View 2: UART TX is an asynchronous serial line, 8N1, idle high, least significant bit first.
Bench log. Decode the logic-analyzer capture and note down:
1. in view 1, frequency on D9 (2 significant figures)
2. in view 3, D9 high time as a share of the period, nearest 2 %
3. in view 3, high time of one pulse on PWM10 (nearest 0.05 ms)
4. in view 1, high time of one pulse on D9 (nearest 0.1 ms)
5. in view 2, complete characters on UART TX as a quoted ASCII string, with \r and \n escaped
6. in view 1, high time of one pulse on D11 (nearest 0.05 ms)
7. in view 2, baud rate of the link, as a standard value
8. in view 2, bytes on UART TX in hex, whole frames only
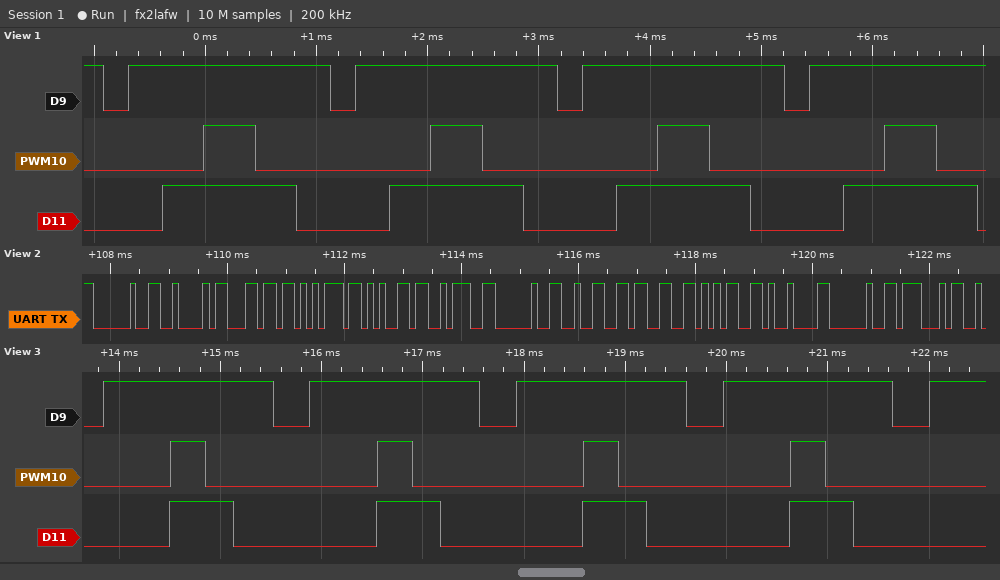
490 Hz
82 %
0.35 ms
1.8 ms
" Blue: 235\t G"
1.20 ms
9600 baud
0x20 0x42 0x6C 0x75 0x65 0x3A 0x20 0x32 0x33 0x35 0x09 0x20 0x47
